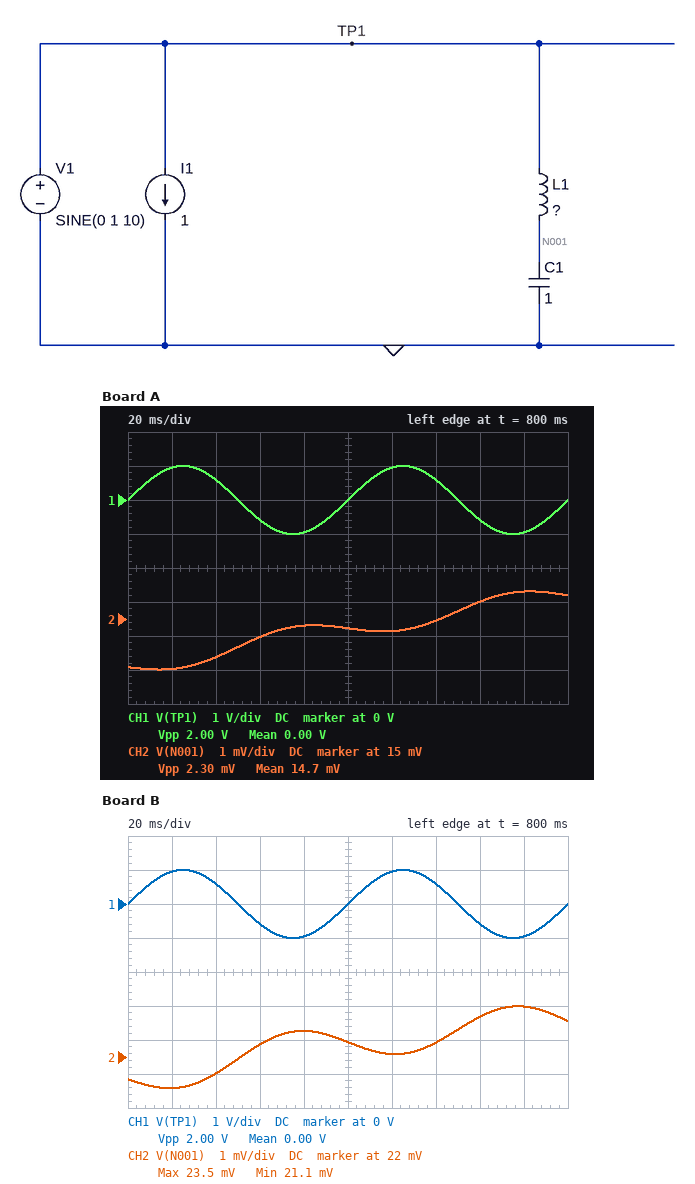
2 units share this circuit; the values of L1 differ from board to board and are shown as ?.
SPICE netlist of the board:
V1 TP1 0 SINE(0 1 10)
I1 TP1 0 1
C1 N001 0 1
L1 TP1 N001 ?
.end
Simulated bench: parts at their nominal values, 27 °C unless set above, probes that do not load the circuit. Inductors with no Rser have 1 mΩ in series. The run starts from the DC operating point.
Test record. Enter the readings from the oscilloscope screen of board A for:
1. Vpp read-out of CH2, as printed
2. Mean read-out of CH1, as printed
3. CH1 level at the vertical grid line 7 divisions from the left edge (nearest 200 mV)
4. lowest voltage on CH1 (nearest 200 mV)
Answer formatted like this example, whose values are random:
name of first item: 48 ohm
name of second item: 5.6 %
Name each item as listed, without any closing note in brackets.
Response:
Vpp read-out of CH2, as printed: 2.30 mV
Mean read-out of CH1, as printed: 0.00 V
CH1 level at the vertical grid line 7 divisions from the left edge: 600 mV
lowest voltage on CH1: -1.0 V
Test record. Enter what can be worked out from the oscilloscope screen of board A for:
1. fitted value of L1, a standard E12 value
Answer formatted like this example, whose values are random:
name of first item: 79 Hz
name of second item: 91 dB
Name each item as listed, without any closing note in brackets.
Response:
fitted value of L1, a standard E12 value: 820 mH
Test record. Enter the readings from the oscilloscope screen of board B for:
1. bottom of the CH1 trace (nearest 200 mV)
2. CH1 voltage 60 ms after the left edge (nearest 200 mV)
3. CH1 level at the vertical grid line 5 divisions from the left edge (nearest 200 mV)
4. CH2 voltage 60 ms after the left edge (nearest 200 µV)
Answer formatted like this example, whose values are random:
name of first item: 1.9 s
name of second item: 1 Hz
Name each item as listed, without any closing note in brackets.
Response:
bottom of the CH1 trace: -1.0 V
CH1 voltage 60 ms after the left edge: -600 mV
CH1 level at the vertical grid line 5 divisions from the left edge: 0 V
CH2 voltage 60 ms after the left edge: 22.4 mV
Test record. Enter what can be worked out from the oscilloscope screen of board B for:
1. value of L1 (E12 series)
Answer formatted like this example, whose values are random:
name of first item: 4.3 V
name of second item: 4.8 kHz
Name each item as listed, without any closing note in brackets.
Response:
value of L1: 470 mH
